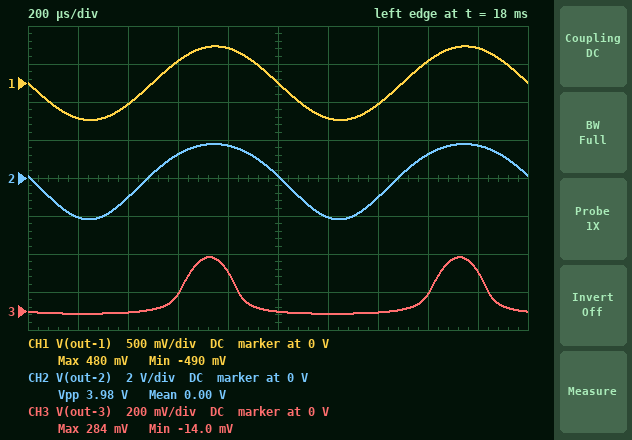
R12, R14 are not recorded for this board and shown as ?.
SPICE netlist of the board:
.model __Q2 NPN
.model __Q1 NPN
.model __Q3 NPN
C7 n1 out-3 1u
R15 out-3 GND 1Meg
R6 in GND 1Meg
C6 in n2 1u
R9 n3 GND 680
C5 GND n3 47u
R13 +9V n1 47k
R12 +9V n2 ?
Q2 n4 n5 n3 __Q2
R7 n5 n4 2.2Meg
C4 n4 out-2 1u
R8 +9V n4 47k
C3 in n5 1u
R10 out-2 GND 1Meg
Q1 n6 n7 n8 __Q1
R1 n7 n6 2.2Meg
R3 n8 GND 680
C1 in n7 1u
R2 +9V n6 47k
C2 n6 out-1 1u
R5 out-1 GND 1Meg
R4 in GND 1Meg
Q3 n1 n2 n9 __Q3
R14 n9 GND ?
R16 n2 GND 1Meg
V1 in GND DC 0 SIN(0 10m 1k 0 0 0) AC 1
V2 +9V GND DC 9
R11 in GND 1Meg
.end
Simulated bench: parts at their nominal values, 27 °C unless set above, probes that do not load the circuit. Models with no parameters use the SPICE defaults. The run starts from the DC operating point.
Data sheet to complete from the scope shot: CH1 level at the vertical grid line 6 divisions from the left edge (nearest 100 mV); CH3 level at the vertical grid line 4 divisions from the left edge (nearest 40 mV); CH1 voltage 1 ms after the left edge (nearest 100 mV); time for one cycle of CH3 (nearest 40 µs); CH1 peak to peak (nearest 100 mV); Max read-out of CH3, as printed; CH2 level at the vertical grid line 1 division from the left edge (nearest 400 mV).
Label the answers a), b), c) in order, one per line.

a) -500 mV
b) 200 mV
c) 0 V
d) 1.00 ms
e) 1.0 V
f) 284 mV
g) -2.0 V
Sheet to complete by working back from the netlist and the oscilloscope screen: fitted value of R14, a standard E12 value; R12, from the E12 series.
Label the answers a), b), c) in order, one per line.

a) 470 Ω
b) 680 kΩ
